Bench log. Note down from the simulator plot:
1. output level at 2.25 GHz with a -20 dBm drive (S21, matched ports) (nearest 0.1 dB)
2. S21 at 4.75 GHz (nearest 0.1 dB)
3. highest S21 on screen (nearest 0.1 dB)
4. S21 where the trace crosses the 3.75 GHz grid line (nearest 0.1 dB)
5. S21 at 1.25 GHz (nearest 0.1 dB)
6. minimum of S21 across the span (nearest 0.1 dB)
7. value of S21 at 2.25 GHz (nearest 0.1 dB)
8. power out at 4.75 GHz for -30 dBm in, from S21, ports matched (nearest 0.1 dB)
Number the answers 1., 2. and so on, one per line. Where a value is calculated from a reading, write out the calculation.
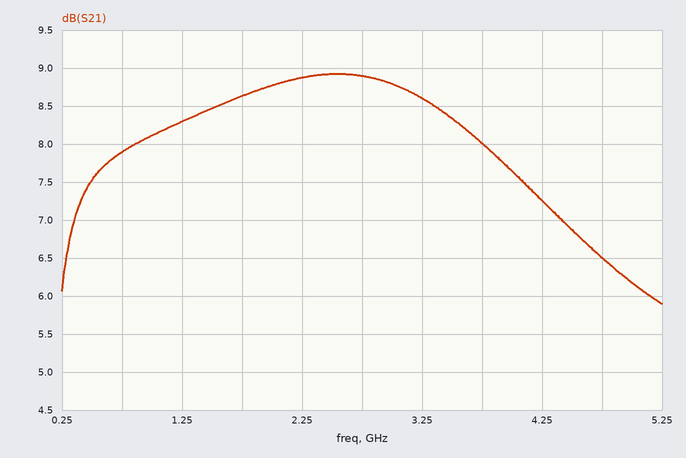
1. -20 dBm + (8.9 dB) = -11.1 dBm
2. 6.5 dB
3. 8.9 dB
4. 8.0 dB
5. 8.3 dB
6. 5.9 dB
7. 8.9 dB
8. -30 dBm + (6.5 dB) = -23.5 dBm
